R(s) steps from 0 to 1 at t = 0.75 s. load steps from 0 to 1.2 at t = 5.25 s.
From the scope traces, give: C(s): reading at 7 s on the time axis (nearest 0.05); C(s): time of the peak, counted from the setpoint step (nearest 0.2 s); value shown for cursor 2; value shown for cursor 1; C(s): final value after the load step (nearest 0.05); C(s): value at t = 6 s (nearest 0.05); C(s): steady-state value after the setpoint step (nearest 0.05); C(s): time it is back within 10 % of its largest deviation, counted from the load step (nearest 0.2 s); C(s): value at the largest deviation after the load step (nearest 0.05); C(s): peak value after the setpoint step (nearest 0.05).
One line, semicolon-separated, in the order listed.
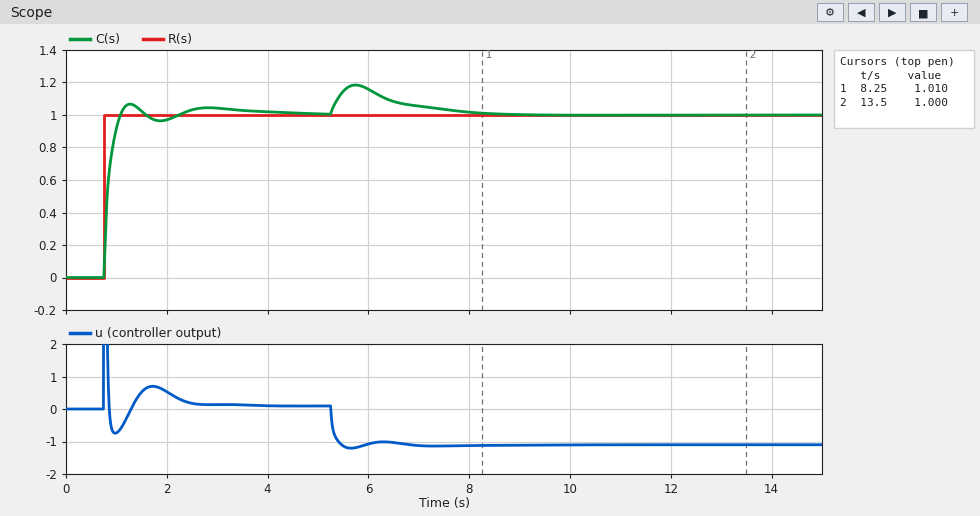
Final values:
1.05; 0.6 s; 1.000; 1.010; 1.00; 1.15; 1.00; 2.8 s; 1.20; 1.05
